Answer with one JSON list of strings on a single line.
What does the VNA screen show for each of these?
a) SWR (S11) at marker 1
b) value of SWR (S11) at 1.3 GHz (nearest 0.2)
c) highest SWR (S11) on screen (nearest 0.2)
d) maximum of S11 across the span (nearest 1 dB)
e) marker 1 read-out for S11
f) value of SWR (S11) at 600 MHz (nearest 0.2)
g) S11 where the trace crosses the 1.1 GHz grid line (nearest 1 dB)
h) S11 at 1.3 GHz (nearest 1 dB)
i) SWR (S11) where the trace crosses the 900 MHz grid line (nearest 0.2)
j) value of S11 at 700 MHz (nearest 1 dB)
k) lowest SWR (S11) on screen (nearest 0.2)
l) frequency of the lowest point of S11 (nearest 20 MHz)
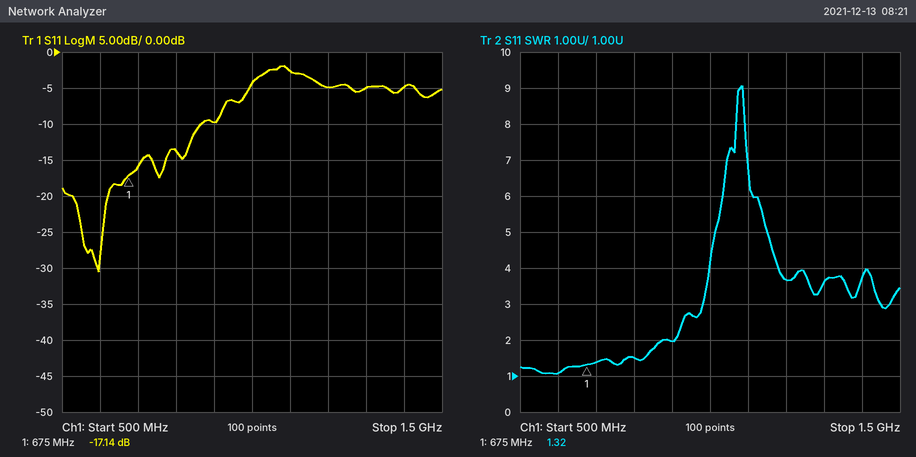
["1.32", "3.6", "9.0", "-2 dB", "-17.14 dB", "1.0", "-3 dB", "-5 dB", "2.0", "-16 dB", "1.0", "600 MHz"]
